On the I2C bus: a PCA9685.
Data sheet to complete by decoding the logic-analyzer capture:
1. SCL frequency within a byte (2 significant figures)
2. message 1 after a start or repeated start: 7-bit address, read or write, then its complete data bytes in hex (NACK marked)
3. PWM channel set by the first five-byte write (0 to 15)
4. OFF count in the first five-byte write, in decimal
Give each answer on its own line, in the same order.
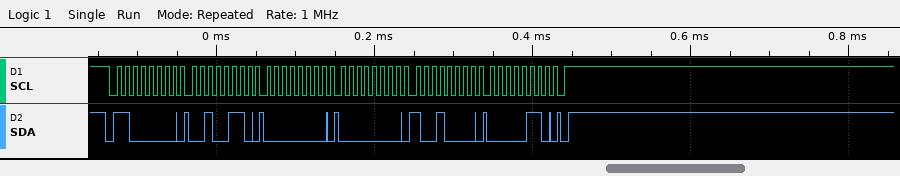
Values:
100 kHz
0x60 write: 26 00 00 90 06
8
1680
